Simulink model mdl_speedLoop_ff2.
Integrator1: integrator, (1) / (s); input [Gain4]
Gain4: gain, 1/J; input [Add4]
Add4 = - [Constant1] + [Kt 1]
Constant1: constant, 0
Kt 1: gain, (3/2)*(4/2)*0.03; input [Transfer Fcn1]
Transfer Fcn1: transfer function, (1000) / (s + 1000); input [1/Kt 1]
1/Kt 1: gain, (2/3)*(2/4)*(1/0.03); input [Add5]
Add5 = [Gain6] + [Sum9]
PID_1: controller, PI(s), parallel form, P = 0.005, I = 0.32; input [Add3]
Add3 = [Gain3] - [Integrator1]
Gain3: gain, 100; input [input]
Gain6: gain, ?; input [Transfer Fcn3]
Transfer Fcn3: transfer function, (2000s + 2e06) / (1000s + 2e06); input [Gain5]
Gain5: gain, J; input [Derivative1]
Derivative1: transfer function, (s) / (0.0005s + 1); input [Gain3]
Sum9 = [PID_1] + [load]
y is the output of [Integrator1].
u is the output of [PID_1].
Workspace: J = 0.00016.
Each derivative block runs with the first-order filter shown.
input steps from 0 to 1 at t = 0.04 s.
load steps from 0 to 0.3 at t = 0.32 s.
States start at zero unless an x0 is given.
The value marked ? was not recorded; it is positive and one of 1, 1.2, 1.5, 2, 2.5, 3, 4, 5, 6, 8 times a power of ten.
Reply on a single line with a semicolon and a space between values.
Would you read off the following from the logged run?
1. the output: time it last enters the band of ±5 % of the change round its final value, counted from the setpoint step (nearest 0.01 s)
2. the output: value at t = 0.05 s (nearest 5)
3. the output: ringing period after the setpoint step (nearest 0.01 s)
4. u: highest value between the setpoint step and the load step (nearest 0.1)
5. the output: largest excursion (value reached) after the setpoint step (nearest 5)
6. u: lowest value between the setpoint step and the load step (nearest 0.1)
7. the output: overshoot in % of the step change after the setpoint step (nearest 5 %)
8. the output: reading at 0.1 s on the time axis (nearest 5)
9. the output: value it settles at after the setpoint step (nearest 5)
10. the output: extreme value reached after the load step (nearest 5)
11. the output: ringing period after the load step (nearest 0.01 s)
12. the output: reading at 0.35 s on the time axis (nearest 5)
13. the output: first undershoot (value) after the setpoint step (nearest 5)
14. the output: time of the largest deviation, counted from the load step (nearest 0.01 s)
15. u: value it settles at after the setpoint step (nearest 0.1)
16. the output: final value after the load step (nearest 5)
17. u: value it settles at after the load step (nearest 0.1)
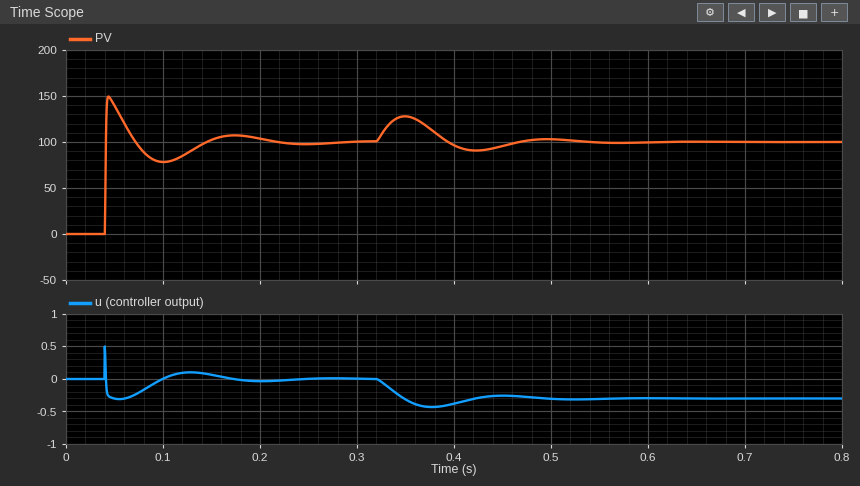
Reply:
0.15 s; 140; 0.13 s; 0.5; 150; -0.3; 50 %; 80; 100; 130; 0.15 s; 130; 80; 0.03 s; 0.0; 100; -0.3
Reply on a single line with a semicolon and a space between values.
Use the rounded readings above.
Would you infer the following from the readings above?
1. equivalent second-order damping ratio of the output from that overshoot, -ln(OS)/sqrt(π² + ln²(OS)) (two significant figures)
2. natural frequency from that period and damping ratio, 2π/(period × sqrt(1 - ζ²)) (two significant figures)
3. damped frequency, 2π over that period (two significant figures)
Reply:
0.22; 50 rad/s; 48 rad/s
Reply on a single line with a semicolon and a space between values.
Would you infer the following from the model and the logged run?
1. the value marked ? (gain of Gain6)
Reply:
1.5
